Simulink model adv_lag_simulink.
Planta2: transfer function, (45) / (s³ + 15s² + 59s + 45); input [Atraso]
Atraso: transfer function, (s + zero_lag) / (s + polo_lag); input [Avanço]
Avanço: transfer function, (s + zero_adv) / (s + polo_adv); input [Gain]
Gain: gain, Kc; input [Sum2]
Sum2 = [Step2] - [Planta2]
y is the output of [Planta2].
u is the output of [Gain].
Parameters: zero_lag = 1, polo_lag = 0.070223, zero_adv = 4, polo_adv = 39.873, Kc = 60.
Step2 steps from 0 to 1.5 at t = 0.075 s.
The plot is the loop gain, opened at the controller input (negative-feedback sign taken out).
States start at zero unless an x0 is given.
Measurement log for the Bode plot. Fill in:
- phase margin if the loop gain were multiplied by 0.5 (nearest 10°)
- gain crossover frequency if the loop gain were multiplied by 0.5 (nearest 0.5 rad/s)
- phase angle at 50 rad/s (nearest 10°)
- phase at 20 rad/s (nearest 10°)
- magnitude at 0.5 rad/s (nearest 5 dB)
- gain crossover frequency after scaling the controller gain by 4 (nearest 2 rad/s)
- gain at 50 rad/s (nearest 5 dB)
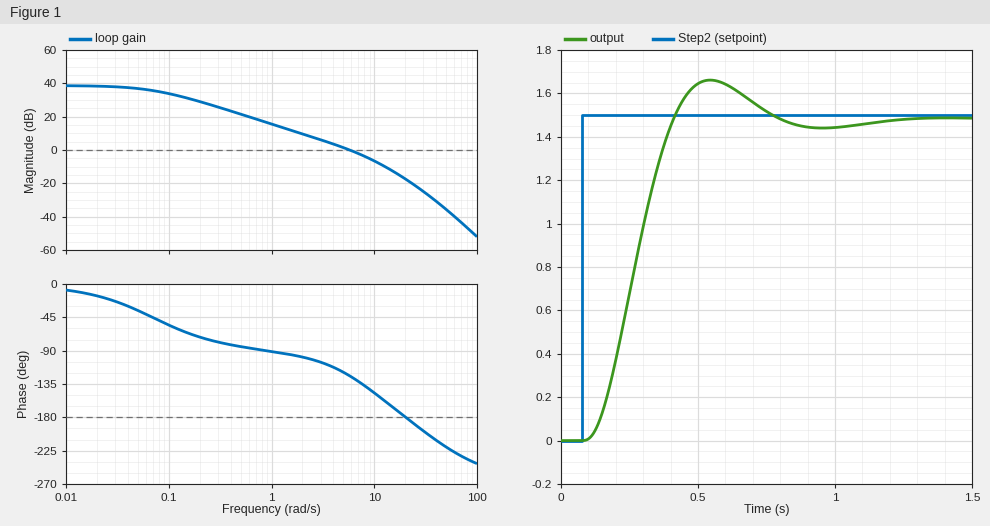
70°
3.0 rad/s
-220°
-180°
20 dB
14 rad/s
-35 dB
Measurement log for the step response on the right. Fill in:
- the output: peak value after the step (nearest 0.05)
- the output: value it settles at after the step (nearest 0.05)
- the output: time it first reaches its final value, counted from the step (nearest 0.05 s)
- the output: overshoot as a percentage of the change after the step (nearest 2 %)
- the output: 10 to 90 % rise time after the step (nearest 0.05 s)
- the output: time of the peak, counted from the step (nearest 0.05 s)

1.65
1.50
0.35 s
12 %
0.20 s
0.45 s
